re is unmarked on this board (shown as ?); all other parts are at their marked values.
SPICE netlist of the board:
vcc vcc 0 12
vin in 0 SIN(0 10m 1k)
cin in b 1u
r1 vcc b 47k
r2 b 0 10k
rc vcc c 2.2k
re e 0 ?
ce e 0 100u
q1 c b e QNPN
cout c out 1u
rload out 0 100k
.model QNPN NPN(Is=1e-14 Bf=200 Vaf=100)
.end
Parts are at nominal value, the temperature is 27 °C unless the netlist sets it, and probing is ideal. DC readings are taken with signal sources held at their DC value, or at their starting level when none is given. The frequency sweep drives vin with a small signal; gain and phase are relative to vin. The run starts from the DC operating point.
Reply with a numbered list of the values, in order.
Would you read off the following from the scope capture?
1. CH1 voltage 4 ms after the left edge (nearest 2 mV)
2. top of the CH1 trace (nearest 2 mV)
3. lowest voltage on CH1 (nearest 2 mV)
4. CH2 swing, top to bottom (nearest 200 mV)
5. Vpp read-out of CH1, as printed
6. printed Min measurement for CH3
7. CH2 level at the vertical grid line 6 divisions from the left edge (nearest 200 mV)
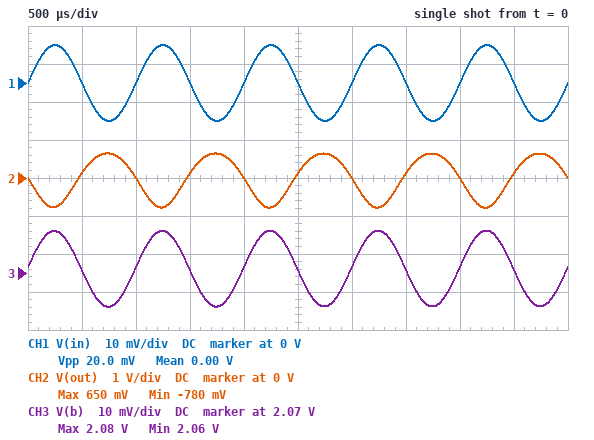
1. 0 V
2. 10 mV
3. -10 mV
4. 1.4 V
5. 20.0 mV
6. 2.06 V
7. 0 V
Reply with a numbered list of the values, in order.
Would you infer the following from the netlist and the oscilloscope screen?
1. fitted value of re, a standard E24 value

1. 1.6 kΩ
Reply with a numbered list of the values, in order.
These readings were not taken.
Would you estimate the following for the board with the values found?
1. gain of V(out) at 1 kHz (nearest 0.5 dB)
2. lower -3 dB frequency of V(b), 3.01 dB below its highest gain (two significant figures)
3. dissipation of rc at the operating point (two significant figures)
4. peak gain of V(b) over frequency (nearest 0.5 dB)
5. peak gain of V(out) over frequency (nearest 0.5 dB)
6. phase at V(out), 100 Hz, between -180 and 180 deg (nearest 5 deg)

1. 37.0 dB
2. 47 Hz
3. 1.7 mW
4. 0 dB
5. 37.0 dB
6. -130 deg
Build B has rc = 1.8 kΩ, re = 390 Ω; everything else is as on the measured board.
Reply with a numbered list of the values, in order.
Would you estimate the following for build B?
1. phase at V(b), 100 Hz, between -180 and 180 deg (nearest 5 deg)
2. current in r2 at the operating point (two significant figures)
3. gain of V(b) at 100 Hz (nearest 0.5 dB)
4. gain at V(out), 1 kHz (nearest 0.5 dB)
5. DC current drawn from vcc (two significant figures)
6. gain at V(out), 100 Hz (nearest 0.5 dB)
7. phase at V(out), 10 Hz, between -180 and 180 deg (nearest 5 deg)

1. 15 deg
2. 200 µA
3. -3.0 dB
4. 46.0 dB
5. 3.5 mA
6. 36.5 dB
7. -50 deg
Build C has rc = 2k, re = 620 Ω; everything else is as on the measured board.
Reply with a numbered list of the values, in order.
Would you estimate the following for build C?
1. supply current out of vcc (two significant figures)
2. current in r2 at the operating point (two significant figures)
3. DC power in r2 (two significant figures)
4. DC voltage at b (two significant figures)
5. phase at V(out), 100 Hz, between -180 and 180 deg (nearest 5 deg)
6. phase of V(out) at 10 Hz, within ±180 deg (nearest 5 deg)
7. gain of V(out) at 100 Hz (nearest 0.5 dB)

1. 2.4 mA
2. 200 µA
3. 410 µW
4. 2.0 V
5. -110 deg
6. -45 deg
7. 37.0 dB
